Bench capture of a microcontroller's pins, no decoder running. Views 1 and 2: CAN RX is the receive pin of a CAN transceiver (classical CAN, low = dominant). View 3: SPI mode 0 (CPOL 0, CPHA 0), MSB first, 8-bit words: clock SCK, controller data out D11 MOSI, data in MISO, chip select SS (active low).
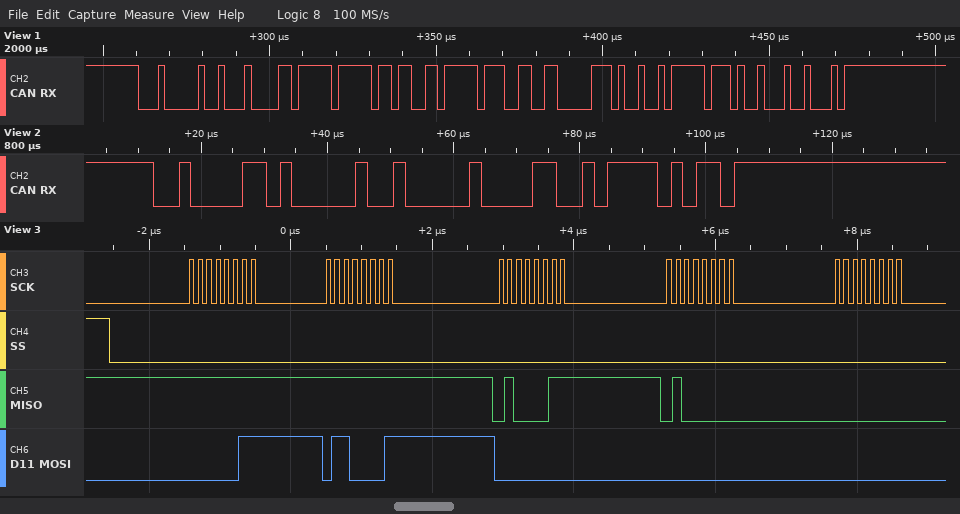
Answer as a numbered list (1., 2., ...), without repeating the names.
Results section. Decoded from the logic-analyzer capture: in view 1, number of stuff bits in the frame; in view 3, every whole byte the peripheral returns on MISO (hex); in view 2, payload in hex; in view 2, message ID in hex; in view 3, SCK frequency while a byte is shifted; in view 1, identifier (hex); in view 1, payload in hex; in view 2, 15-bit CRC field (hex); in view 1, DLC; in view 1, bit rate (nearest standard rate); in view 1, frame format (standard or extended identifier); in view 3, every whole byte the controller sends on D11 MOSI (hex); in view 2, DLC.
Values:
1. 6
2. FF FF 43 40 00
3. 00
4. 0x21A
5. 8 MHz
6. 0x101
7. 6F FF 66 FF 33 06 92 FF
8. 0x32F5
9. 8
10. 500 kbit/s
11. standard
12. 03 61 00 00 00
13. 1
